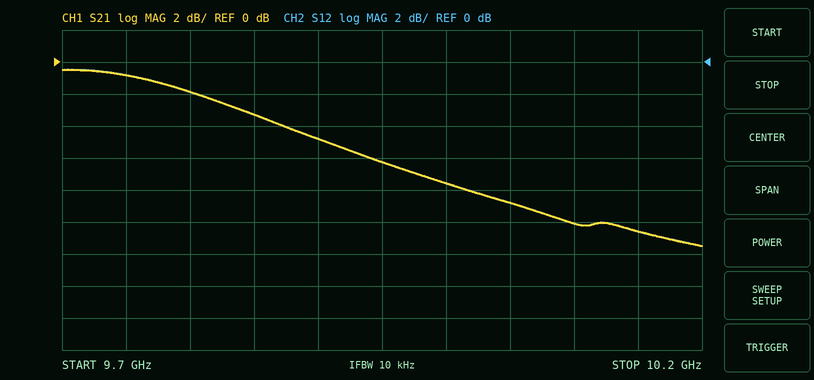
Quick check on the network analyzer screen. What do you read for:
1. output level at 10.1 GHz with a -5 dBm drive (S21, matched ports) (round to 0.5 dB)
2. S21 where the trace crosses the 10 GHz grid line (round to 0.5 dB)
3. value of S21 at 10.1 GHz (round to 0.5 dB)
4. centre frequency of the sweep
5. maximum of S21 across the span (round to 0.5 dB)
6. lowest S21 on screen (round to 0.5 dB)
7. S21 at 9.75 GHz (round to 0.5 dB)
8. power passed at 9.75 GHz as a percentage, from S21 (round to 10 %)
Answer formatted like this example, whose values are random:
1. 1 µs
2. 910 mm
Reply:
1. -15.0 dBm
2. -7.5 dB
3. -10.0 dB
4. 9.95 GHz
5. -0.5 dB
6. -11.5 dB
7. -1.0 dB
8. 80 %
